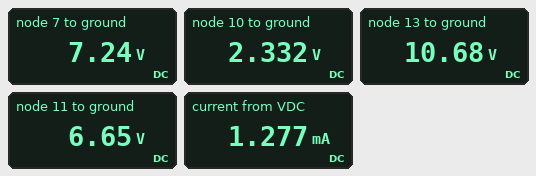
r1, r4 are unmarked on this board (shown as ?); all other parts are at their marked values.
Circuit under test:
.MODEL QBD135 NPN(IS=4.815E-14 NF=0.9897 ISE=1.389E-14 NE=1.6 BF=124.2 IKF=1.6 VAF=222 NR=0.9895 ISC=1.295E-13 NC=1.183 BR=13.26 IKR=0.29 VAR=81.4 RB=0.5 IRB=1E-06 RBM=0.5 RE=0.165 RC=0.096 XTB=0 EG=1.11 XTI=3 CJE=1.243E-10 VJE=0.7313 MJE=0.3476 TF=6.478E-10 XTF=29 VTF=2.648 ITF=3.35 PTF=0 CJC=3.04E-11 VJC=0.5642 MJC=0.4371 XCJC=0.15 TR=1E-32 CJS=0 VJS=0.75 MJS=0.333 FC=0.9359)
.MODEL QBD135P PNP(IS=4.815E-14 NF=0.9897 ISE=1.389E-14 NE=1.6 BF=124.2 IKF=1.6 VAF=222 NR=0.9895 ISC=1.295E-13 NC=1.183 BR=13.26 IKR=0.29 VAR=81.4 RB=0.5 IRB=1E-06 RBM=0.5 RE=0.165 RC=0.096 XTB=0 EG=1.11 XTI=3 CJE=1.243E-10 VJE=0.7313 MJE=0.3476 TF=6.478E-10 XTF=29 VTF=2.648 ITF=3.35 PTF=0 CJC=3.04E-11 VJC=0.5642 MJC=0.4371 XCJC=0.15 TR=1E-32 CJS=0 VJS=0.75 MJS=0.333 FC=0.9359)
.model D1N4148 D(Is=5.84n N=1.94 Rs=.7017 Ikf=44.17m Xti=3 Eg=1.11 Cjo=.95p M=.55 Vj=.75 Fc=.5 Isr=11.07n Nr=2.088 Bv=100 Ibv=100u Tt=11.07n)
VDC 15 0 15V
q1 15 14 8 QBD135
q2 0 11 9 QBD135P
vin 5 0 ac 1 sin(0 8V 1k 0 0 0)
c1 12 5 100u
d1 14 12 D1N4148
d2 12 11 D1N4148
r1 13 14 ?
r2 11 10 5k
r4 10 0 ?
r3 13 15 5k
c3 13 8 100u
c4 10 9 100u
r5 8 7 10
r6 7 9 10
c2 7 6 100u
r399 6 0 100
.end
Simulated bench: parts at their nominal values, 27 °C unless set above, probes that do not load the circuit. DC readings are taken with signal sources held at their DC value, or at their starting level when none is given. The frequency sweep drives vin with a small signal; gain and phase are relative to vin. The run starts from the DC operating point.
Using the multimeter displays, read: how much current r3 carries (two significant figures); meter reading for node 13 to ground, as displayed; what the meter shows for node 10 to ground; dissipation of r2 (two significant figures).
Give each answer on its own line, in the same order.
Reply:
860 µA
10.68 V
2.332 V
3.7 mW
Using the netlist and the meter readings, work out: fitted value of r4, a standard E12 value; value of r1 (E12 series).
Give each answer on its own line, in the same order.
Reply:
2.7 kΩ
3.3 kΩ
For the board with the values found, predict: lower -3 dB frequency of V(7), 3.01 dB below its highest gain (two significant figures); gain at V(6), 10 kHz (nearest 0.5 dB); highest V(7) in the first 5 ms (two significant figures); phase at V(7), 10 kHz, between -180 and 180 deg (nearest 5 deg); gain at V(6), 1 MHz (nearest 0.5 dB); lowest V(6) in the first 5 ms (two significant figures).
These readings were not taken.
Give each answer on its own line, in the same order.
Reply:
340 mHz
-3.0 dB
14 V
0 deg
-3.0 dB
-6.6 V
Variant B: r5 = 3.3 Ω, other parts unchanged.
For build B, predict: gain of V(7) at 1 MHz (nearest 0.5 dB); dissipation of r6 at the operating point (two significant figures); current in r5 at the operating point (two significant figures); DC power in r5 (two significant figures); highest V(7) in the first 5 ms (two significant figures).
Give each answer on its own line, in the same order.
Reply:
-2.5 dB
1.9 µW
440 µA
630 nW
15 V
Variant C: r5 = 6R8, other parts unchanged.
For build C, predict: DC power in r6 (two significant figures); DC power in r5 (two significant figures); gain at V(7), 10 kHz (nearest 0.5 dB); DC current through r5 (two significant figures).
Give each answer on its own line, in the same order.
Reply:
1.8 µW
1.2 µW
-2.5 dB
430 µA
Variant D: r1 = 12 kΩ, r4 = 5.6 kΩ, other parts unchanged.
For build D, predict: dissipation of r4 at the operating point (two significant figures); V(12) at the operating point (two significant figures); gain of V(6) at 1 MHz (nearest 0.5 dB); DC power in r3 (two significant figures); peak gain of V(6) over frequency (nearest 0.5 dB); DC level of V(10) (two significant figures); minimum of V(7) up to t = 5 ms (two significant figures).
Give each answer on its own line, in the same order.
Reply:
1.4 mW
5.9 V
-6.0 dB
1.3 mW
-1.5 dB
2.8 V
710 mV
